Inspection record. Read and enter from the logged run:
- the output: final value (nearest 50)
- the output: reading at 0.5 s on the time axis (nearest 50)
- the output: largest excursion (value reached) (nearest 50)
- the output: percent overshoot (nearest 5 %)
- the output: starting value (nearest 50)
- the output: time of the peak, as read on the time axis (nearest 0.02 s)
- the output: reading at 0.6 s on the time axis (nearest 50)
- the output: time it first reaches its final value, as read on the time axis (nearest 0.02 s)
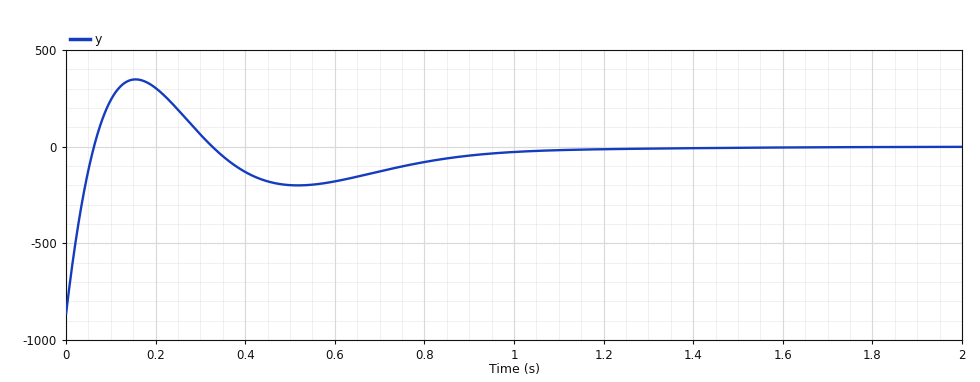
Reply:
0
-200
350
40 %
-850
0.16 s
-200
0.06 s
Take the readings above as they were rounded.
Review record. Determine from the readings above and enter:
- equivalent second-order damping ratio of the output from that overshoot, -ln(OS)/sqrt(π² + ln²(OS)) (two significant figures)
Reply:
0.28
